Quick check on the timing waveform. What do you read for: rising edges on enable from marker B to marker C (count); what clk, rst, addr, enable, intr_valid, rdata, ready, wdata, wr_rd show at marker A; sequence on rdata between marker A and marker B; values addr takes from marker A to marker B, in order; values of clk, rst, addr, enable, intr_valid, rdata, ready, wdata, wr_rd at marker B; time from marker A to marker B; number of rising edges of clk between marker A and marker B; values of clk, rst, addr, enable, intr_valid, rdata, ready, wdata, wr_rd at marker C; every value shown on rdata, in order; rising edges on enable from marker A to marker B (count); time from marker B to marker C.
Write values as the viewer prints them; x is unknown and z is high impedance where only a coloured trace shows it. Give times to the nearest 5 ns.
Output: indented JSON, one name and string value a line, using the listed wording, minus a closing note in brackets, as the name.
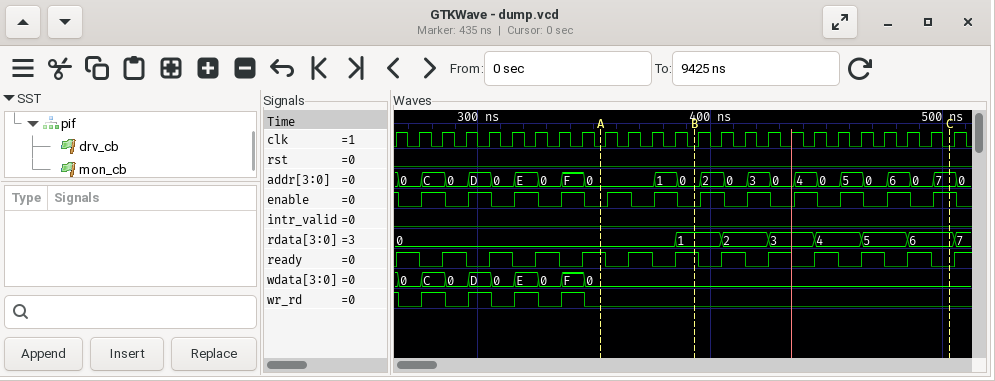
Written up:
{
  "rising edges on enable from marker B to marker C": "6",
  "what clk, rst, addr, enable, intr_valid, rdata, ready, wdata, wr_rd show at marker A": "clk=0, rst=0, addr=0, enable=0, intr_valid=0, rdata=0, ready=1, wdata=0, wr_rd=0",
  "sequence on rdata between marker A and marker B": "0, 1",
  "values addr takes from marker A to marker B, in order": "0, 1, 0",
  "values of clk, rst, addr, enable, intr_valid, rdata, ready, wdata, wr_rd at marker B": "clk=0, rst=0, addr=0, enable=0, intr_valid=0, rdata=1, ready=1, wdata=0, wr_rd=0",
  "time from marker A to marker B": "40 ns",
  "number of rising edges of clk between marker A and marker B": "4",
  "values of clk, rst, addr, enable, intr_valid, rdata, ready, wdata, wr_rd at marker C": "clk=0, rst=0, addr=7, enable=1, intr_valid=0, rdata=6, ready=0, wdata=0, wr_rd=0",
  "every value shown on rdata, in order": "0, 1, 2, 3, 4, 5, 6, 7",
  "rising edges on enable from marker A to marker B": "2",
  "time from marker B to marker C": "110 ns"
}
